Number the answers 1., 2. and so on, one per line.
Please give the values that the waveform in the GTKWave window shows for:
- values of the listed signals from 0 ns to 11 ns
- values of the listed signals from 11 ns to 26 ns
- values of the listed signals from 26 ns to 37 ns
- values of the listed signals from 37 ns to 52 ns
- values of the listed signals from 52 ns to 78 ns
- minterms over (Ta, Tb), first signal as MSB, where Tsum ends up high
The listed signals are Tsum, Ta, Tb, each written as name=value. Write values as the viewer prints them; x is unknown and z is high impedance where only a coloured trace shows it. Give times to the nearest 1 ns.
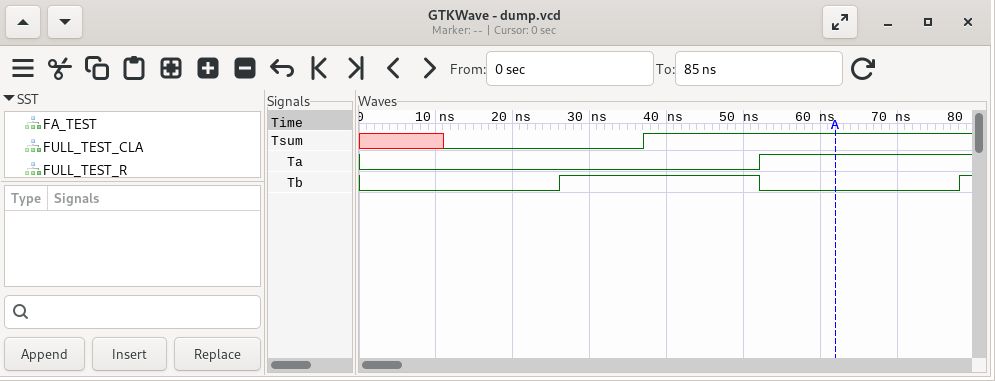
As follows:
1. Tsum=x, Ta=0, Tb=0
2. Tsum=0, Ta=0, Tb=0
3. Tsum=0, Ta=0, Tb=1
4. Tsum=1, Ta=0, Tb=1
5. Tsum=1, Ta=1, Tb=0
6. 1, 2, 3
